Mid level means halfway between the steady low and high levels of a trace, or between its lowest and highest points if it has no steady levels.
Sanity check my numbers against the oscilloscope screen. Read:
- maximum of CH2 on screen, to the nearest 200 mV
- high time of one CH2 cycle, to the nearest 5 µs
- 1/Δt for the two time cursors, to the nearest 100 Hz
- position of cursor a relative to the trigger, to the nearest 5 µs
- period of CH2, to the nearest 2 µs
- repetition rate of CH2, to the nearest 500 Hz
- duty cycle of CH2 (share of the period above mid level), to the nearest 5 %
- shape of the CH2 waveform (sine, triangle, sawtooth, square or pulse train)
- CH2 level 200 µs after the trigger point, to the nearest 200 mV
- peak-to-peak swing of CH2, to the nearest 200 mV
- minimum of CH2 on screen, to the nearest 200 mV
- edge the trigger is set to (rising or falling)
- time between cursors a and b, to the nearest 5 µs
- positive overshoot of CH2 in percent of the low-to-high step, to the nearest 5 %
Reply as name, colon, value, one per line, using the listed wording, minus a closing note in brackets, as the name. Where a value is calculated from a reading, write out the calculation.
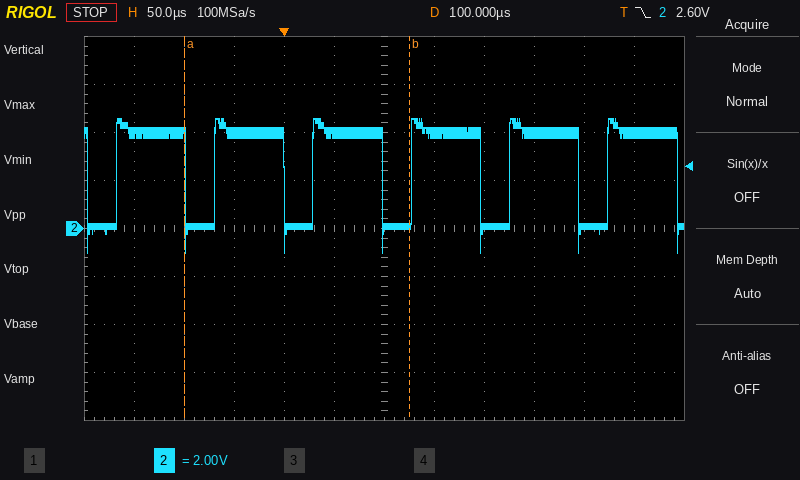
maximum of CH2 on screen, to the nearest 200 mV: 4.6 V
high time of one CH2 cycle, to the nearest 5 µs: 70 µs
1/Δt for the two time cursors, to the nearest 100 Hz: 1 / 225 µs ≈ 4.4 kHz
position of cursor a relative to the trigger, to the nearest 5 µs: -100 µs
period of CH2, to the nearest 2 µs: 98 µs
repetition rate of CH2, to the nearest 500 Hz: 1 / 98 µs ≈ 10.2 kHz, so 10.0 kHz to the nearest 500 Hz
duty cycle of CH2 (share of the period above mid level), to the nearest 5 %: 70 µs / 98 µs ≈ 71.4 %, so 70 % to the nearest 5 %
shape of the CH2 waveform: pulse train
CH2 level 200 µs after the trigger point, to the nearest 200 mV: 0.0 V
peak-to-peak swing of CH2, to the nearest 200 mV: 4.6 V − (-1.0 V) = 5.6 V
minimum of CH2 on screen, to the nearest 200 mV: -1.0 V
edge the trigger is set to: falling
time between cursors a and b, to the nearest 5 µs: 225 µs
positive overshoot of CH2 in percent of the low-to-high step, to the nearest 5 %: 15 %
